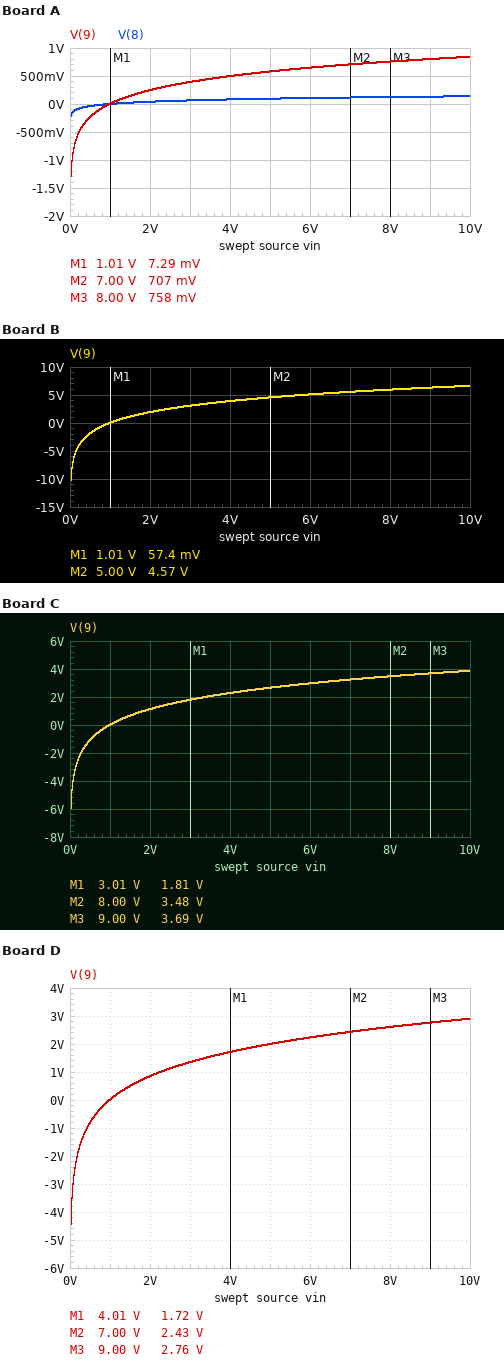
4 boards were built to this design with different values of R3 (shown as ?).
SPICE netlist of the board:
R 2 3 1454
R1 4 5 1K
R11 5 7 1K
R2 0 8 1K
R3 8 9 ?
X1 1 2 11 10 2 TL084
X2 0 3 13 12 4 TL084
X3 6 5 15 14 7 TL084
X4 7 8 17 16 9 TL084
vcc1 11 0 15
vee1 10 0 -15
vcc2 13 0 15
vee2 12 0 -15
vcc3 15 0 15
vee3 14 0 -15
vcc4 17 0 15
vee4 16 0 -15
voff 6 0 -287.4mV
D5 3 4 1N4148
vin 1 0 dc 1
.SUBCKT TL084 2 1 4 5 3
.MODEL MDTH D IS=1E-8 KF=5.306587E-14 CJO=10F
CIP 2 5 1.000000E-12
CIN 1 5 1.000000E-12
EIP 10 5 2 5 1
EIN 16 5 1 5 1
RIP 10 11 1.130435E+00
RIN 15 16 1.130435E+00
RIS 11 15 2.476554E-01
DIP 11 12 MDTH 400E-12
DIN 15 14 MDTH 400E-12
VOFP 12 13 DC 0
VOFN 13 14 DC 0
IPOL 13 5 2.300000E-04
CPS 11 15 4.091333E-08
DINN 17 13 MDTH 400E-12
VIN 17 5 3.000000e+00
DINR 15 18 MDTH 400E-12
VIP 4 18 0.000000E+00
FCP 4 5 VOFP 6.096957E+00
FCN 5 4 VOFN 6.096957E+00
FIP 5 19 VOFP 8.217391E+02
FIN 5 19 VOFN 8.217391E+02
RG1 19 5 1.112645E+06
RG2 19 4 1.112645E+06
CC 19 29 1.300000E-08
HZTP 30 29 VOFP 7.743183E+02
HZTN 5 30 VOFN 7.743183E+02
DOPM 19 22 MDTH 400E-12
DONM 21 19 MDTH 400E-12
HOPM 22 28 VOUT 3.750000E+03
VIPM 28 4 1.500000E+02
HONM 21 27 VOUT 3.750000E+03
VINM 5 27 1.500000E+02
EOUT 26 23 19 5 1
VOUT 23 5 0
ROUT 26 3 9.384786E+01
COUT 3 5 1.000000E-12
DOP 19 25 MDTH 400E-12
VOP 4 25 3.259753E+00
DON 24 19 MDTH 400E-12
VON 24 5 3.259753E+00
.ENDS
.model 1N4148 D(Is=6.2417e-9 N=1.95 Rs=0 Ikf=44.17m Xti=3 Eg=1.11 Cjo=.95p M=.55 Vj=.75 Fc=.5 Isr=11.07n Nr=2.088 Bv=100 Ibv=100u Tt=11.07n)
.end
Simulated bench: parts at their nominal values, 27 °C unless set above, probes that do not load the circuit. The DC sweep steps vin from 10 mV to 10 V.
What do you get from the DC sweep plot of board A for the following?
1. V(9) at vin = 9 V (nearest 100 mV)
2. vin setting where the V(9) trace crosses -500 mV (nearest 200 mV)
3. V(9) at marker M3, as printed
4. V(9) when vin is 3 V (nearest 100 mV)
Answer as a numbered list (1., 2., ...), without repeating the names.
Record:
1. 800 mV
2. 200 mV
3. 758 mV
4. 400 mV
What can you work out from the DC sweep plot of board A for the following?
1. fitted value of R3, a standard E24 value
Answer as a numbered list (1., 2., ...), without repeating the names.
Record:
1. 5.1 kΩ
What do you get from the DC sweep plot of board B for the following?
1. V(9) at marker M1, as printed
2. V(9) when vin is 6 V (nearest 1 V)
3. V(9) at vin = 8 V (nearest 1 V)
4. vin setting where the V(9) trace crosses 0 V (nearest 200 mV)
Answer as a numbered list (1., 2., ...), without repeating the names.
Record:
1. 57.4 mV
2. 5 V
3. 6 V
4. 1.0 V
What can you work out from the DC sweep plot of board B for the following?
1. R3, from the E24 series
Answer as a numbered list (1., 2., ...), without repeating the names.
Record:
1. 47 kΩ
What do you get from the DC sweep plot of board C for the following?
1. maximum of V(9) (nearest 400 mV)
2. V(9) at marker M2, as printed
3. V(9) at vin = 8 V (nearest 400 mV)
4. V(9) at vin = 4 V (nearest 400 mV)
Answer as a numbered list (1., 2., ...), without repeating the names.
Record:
1. 4.0 V
2. 3.48 V
3. 3.6 V
4. 2.4 V
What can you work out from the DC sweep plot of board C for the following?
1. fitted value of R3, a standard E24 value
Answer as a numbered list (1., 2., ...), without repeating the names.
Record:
1. 27 kΩ
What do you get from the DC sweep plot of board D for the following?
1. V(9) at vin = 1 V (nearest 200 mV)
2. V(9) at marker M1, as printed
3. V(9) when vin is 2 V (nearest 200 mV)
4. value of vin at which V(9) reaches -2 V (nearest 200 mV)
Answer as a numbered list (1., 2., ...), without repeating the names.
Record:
1. 0 V
2. 1.72 V
3. 800 mV
4. 200 mV
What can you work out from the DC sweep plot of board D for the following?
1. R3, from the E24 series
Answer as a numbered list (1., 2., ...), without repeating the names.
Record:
1. 20 kΩ
